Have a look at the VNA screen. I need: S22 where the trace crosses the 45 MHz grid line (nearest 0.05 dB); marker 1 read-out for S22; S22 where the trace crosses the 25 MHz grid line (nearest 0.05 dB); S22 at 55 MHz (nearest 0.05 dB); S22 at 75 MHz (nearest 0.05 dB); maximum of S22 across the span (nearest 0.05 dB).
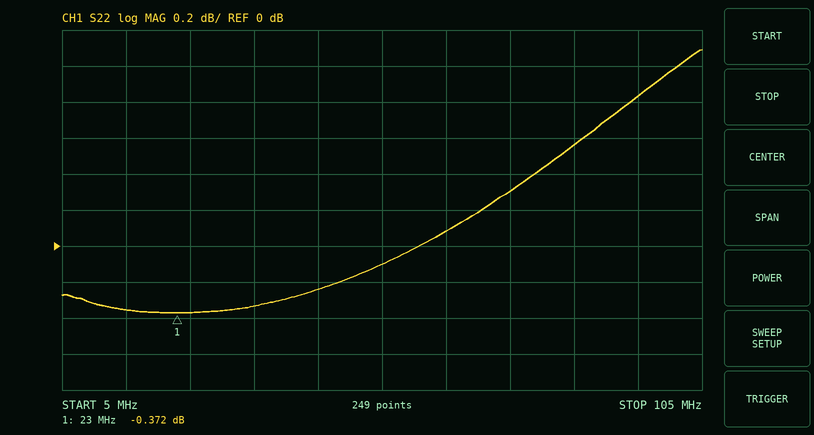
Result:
-0.25 dB
-0.372 dB
-0.35 dB
-0.10 dB
0.30 dB
1.10 dB
